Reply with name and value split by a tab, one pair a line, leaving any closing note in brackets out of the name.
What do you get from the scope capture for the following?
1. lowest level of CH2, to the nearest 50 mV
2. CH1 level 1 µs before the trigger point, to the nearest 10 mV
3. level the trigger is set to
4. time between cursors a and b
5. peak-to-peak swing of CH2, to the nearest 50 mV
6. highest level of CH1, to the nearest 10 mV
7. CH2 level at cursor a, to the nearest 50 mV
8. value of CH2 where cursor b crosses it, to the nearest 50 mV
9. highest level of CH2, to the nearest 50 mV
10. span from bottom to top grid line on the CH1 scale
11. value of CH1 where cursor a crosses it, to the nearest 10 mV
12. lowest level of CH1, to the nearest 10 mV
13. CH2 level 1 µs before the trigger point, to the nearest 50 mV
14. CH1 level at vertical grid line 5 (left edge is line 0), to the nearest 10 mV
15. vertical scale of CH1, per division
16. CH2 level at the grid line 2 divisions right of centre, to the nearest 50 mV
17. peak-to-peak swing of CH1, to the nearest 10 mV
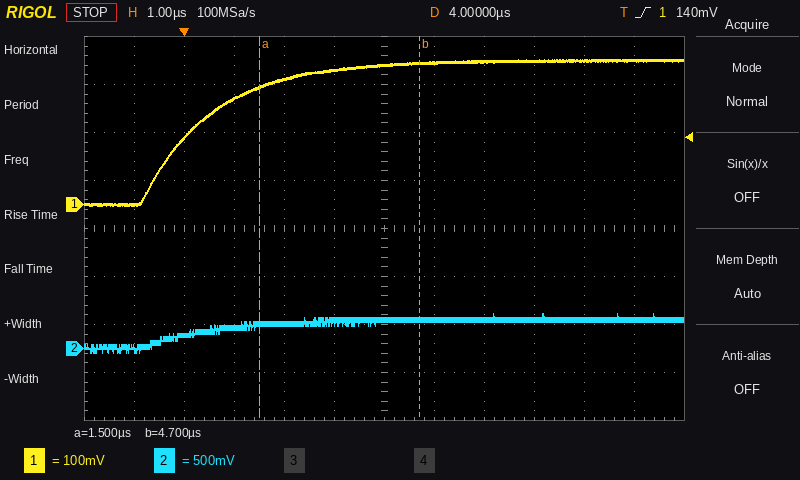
lowest level of CH2, to the nearest 50 mV	-50 mV
CH1 level 1 µs before the trigger point, to the nearest 10 mV	0 mV
level the trigger is set to	140 mV
time between cursors a and b	3.2 µs
peak-to-peak swing of CH2, to the nearest 50 mV	400 mV
highest level of CH1, to the nearest 10 mV	300 mV
CH2 level at cursor a, to the nearest 50 mV	250 mV
value of CH2 where cursor b crosses it, to the nearest 50 mV	300 mV
highest level of CH2, to the nearest 50 mV	350 mV
span from bottom to top grid line on the CH1 scale	800 mV
value of CH1 where cursor a crosses it, to the nearest 10 mV	240 mV
lowest level of CH1, to the nearest 10 mV	0 mV
CH2 level 1 µs before the trigger point, to the nearest 50 mV	0 mV
CH1 level at vertical grid line 5 (left edge is line 0), to the nearest 10 mV	280 mV
vertical scale of CH1, per division	100 mV
CH2 level at the grid line 2 divisions right of centre, to the nearest 50 mV	300 mV
peak-to-peak swing of CH1, to the nearest 10 mV	300 mV
